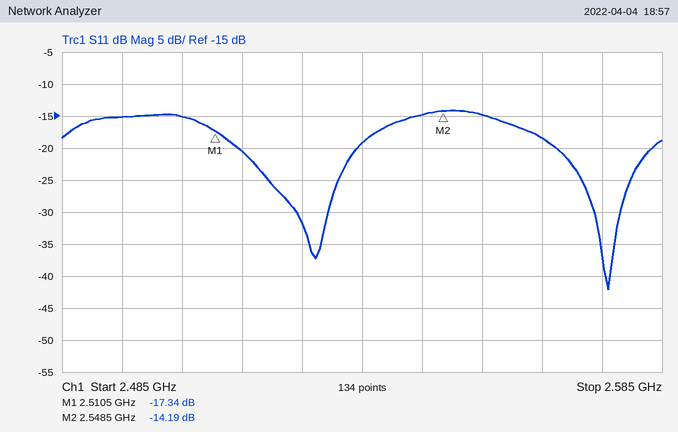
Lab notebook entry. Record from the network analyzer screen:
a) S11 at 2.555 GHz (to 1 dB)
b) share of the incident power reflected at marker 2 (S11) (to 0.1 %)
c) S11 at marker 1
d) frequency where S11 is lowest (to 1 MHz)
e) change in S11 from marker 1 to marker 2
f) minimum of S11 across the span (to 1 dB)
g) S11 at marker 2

-15 dB
3.8 %
-17.34 dB
2.576 GHz
3.15 dB
-42 dB
-14.19 dB
